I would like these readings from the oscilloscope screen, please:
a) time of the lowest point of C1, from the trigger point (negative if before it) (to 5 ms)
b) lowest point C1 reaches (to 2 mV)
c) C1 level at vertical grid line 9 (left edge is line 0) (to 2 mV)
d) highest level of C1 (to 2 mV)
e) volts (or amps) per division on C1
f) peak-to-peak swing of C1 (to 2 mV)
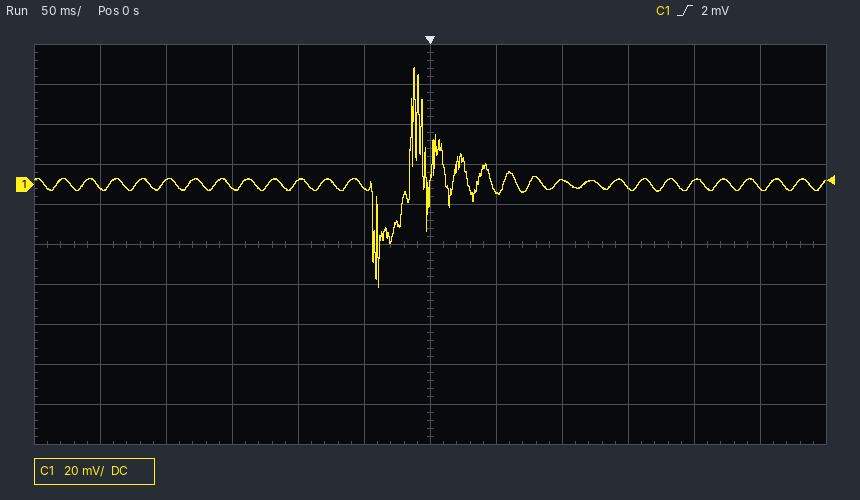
-40 ms
-52 mV
-2 mV
58 mV
20 mV
110 mV
